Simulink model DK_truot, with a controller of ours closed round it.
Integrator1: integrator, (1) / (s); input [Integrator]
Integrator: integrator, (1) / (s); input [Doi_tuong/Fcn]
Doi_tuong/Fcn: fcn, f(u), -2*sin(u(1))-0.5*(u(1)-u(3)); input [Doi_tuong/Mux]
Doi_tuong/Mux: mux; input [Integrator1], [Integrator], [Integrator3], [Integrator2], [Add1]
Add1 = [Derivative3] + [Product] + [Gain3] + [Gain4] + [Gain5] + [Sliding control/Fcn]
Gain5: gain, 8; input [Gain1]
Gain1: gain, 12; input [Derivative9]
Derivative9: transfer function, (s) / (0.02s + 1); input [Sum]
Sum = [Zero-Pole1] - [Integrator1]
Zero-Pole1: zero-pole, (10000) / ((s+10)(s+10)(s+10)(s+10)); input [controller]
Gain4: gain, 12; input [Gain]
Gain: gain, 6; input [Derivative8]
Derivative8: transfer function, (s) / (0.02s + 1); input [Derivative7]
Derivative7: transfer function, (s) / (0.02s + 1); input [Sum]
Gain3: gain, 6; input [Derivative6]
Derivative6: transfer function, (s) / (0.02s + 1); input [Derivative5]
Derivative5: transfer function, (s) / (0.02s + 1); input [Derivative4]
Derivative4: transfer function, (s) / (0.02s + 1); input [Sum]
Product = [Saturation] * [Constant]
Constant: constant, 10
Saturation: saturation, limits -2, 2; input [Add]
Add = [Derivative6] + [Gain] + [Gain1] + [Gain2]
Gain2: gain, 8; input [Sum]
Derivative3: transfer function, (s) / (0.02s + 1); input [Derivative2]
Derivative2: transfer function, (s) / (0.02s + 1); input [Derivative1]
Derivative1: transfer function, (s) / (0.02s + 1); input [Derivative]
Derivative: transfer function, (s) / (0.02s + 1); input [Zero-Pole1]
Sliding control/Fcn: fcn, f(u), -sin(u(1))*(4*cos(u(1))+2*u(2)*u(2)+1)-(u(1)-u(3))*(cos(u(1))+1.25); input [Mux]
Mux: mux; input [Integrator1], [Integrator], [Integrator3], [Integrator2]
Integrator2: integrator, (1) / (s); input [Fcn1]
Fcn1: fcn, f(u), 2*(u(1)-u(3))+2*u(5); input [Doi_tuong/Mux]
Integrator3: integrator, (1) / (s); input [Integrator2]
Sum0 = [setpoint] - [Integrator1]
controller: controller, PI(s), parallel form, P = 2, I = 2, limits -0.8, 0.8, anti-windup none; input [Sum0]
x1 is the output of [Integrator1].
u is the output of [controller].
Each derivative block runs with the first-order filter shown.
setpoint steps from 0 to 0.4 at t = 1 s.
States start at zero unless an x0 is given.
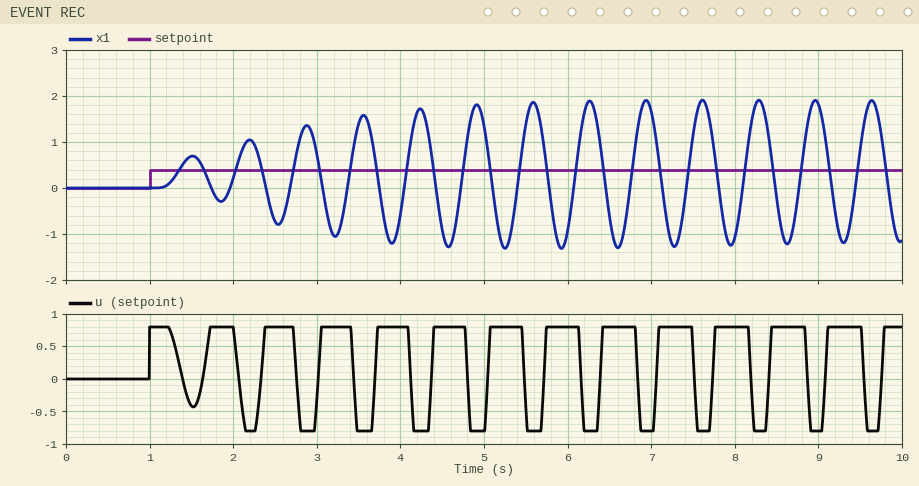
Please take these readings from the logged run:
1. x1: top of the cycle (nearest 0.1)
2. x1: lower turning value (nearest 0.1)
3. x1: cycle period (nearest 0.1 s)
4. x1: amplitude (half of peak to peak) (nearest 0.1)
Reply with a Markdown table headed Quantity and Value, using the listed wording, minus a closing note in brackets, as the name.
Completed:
| Quantity | Value |
|---|---|
| x1: top of the cycle | 1.9 |
| x1: lower turning value | -1.3 |
| x1: cycle period | 0.7 s |
| x1: amplitude (half of peak to peak) | 1.6 |
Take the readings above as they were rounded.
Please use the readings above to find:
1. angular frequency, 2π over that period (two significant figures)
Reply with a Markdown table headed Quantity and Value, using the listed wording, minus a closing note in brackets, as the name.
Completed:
| Quantity | Value |
|---|---|
| angular frequency, 2π over that period | 9.0 rad/s |
